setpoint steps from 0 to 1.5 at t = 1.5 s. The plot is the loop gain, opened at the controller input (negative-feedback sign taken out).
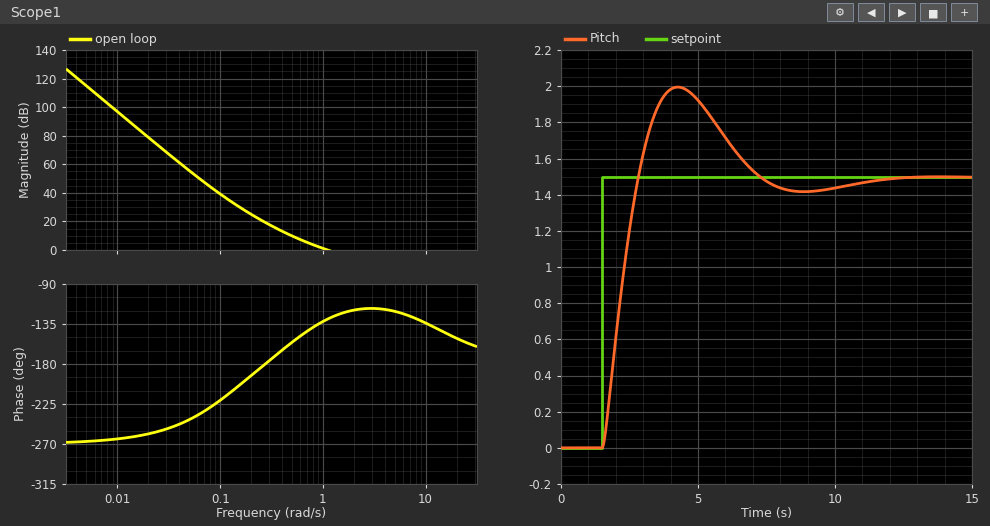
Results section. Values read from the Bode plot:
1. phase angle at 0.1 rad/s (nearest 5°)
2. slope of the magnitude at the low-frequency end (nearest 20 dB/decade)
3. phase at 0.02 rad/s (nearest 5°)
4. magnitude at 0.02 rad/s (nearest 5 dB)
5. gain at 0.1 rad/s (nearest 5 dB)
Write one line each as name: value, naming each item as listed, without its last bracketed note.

phase angle at 0.1 rad/s: -220°
slope of the magnitude at the low-frequency end: -60 dB/decade
phase at 0.02 rad/s: -260°
magnitude at 0.02 rad/s: 80 dB
gain at 0.1 rad/s: 40 dB
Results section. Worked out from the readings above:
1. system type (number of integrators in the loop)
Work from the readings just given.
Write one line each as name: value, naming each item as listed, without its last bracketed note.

system type: 3
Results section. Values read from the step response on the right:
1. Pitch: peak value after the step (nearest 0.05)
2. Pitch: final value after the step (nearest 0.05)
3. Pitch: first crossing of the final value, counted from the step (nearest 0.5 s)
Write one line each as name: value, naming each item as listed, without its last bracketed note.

Pitch: peak value after the step: 2.00
Pitch: final value after the step: 1.50
Pitch: first crossing of the final value, counted from the step: 1.5 s
